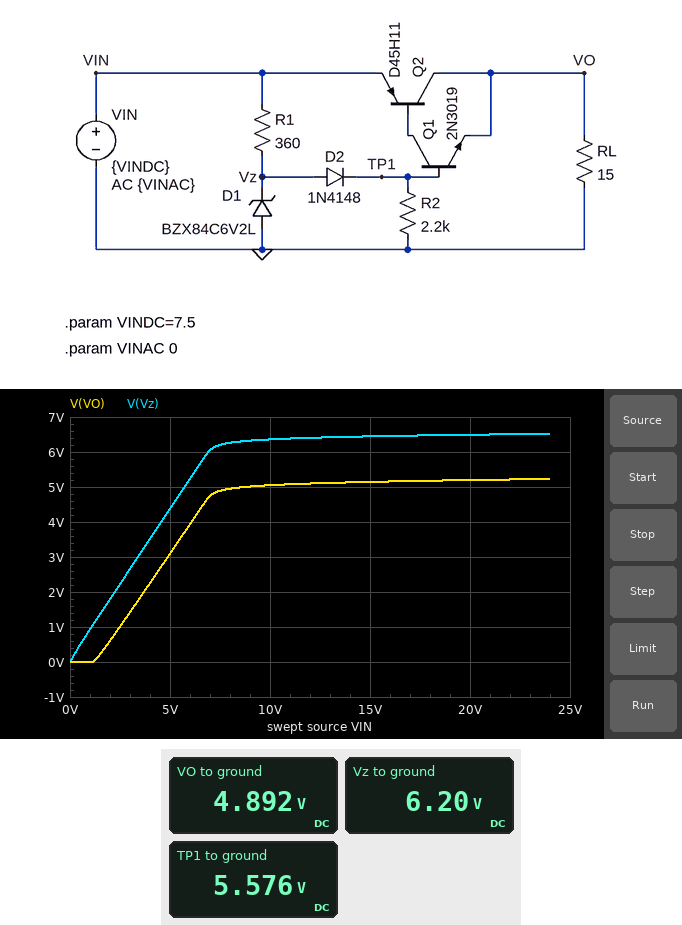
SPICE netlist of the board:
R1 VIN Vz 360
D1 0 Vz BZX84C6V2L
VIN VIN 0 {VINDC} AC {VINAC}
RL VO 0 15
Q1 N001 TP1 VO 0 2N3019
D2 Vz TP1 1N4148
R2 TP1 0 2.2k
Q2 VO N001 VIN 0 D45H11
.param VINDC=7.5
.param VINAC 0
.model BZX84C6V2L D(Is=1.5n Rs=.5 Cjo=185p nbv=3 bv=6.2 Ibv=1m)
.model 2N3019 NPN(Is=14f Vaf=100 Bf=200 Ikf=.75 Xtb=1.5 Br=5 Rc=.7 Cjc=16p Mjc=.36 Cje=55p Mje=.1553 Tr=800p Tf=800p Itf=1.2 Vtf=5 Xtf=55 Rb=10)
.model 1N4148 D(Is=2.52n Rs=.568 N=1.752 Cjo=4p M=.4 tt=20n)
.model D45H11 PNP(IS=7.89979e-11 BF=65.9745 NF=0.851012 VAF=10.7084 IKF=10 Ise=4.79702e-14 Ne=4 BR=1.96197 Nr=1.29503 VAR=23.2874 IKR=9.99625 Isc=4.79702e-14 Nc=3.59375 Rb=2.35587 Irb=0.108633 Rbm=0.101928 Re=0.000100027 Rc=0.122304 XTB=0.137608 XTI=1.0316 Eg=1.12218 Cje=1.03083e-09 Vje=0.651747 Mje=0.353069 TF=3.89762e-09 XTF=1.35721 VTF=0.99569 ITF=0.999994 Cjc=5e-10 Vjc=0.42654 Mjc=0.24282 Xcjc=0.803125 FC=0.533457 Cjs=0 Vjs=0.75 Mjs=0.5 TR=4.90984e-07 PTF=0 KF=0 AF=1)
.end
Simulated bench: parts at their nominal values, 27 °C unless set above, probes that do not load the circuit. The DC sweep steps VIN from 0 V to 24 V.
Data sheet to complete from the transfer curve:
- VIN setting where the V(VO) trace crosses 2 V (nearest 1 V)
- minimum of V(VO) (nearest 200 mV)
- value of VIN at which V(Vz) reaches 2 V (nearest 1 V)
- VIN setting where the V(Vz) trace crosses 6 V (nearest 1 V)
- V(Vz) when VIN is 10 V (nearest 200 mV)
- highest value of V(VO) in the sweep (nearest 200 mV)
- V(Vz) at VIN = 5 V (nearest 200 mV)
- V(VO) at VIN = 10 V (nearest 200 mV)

4 V
0 V
2 V
7 V
6.4 V
5.2 V
4.4 V
5.0 V
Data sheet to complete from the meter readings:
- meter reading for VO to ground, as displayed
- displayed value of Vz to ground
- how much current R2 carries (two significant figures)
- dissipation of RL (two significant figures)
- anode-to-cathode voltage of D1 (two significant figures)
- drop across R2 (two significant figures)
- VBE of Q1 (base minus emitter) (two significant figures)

4.892 V
6.20 V
2.5 mA
1.6 W
-6.2 V
5.6 V
680 mV
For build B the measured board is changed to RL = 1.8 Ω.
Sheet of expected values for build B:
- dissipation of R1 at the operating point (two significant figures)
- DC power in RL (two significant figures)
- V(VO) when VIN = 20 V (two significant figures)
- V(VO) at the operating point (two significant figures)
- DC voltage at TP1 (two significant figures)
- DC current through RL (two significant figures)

4.8 mW
13 W
5.1 V
4.8 V
5.6 V
2.7 A
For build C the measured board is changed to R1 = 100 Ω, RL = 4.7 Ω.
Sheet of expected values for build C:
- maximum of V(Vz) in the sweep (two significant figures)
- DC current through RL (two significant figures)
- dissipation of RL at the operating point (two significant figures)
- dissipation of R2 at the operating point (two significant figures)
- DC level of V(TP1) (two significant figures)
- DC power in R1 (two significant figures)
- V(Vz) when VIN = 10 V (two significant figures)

6.7 V
1.1 A
5.4 W
15 mW
5.7 V
13 mW
6.5 V
